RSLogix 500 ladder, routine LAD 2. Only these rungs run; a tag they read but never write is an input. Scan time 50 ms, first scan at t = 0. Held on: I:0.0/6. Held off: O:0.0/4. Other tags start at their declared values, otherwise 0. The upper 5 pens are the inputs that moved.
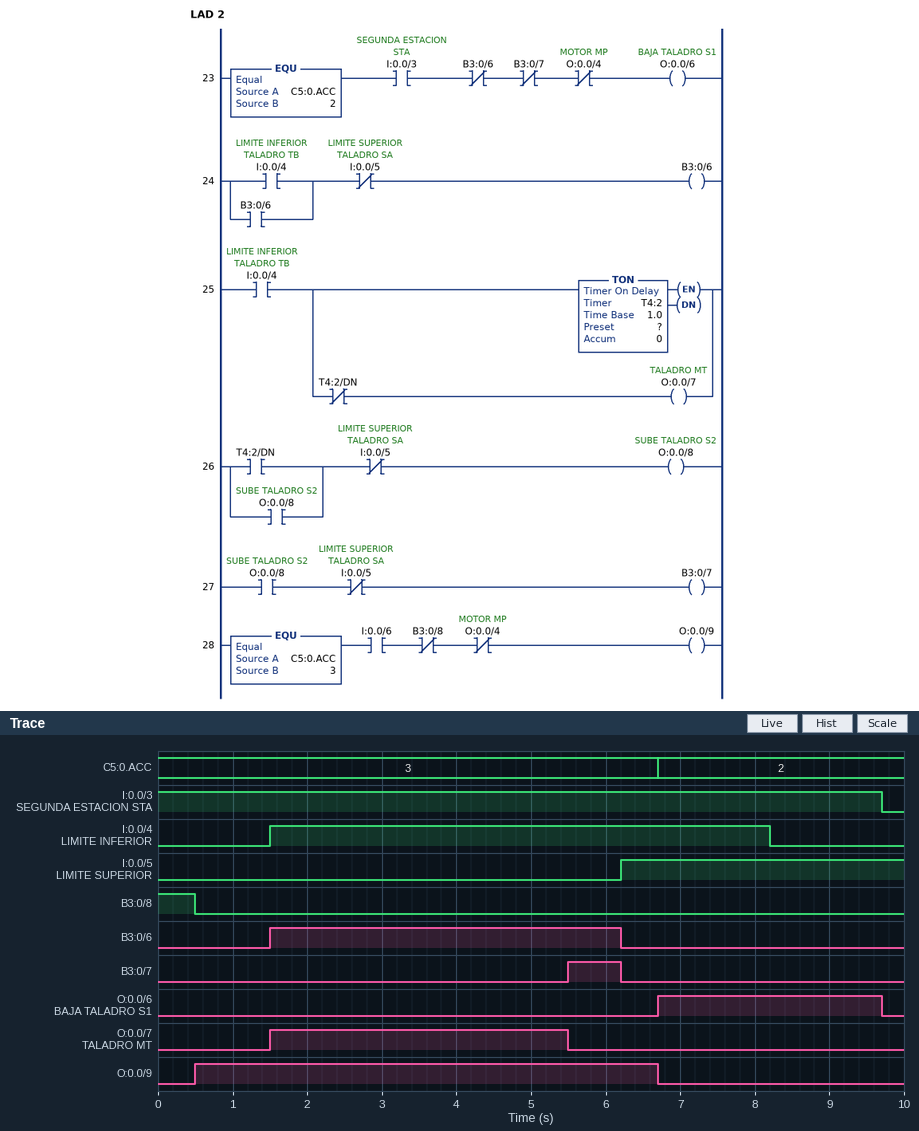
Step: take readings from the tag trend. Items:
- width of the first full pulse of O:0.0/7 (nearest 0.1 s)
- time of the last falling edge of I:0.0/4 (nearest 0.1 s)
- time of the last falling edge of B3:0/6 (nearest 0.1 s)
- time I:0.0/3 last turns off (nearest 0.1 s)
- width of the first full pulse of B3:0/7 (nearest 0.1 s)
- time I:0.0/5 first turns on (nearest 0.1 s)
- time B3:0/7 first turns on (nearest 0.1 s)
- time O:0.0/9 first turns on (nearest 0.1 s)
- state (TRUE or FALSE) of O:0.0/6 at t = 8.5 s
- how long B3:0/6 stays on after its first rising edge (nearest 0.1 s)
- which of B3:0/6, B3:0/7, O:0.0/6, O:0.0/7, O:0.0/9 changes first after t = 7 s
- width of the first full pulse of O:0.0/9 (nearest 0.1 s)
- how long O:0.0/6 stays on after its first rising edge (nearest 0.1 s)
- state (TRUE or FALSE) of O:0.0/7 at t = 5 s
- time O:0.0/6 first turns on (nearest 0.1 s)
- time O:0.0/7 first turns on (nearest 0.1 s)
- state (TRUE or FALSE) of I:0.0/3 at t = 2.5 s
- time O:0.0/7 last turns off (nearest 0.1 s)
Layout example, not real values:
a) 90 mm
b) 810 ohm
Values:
a) 4.0 s
b) 8.2 s
c) 6.2 s
d) 9.7 s
e) 0.7 s
f) 6.2 s
g) 5.5 s
h) 0.5 s
i) TRUE
j) 4.7 s
k) O:0.0/6
l) 6.2 s
m) 3.0 s
n) TRUE
o) 6.7 s
p) 1.5 s
q) TRUE
r) 5.5 s
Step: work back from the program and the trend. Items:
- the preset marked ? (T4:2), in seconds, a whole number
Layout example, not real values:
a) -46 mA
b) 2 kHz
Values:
a) 4 s
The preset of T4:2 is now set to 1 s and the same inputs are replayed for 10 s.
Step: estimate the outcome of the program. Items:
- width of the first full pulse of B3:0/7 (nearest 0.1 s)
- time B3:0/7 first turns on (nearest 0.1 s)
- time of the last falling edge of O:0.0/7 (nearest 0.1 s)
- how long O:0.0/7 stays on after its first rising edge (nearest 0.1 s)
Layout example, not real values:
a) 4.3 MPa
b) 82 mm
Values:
a) 3.7 s
b) 2.5 s
c) 2.5 s
d) 1.0 s
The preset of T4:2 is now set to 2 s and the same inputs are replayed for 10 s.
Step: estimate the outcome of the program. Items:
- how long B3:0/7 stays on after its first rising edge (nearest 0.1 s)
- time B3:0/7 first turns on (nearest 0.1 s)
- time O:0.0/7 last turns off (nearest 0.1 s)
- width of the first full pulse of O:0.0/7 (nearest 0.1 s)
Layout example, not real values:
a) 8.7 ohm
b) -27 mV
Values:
a) 2.7 s
b) 3.5 s
c) 3.5 s
d) 2.0 s
